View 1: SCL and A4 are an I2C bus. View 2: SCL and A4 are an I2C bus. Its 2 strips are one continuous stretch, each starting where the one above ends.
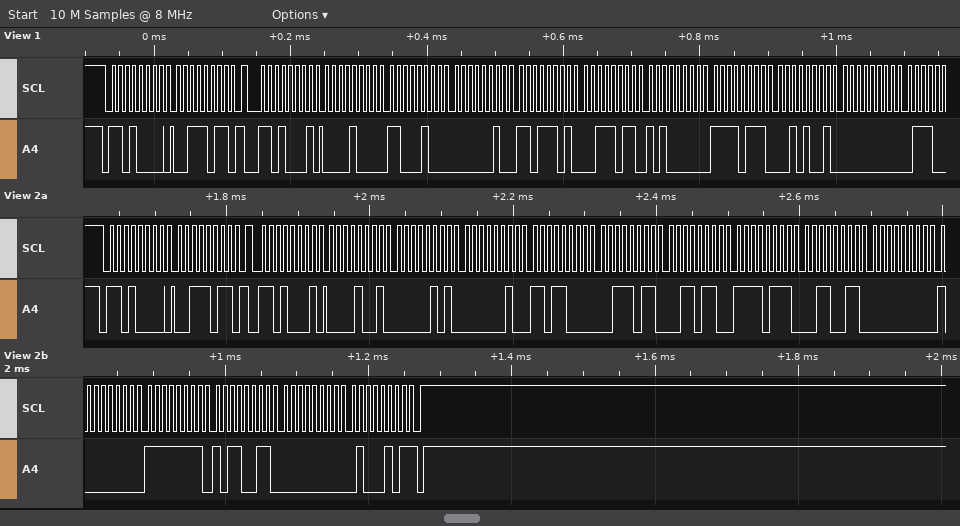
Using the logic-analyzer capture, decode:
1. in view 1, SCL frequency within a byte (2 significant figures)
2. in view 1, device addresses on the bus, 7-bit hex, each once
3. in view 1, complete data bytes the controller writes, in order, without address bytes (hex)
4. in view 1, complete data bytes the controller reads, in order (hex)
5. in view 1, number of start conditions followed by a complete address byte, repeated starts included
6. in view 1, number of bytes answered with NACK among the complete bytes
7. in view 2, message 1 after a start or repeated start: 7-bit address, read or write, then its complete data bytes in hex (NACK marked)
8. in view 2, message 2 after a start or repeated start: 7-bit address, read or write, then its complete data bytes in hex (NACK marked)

100 kHz
0x68
3B
08 C4 02 DD 3B A0 F7 29 00
2
0
0x68 write: 3B
0x68 read: 09 05 02 D8 3B 36 F7 33 00 80 FF B3 00 45 NACK
